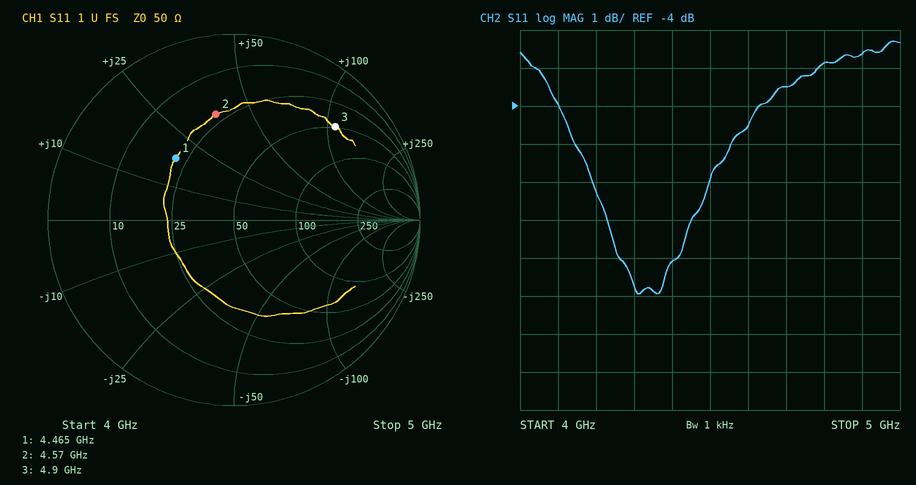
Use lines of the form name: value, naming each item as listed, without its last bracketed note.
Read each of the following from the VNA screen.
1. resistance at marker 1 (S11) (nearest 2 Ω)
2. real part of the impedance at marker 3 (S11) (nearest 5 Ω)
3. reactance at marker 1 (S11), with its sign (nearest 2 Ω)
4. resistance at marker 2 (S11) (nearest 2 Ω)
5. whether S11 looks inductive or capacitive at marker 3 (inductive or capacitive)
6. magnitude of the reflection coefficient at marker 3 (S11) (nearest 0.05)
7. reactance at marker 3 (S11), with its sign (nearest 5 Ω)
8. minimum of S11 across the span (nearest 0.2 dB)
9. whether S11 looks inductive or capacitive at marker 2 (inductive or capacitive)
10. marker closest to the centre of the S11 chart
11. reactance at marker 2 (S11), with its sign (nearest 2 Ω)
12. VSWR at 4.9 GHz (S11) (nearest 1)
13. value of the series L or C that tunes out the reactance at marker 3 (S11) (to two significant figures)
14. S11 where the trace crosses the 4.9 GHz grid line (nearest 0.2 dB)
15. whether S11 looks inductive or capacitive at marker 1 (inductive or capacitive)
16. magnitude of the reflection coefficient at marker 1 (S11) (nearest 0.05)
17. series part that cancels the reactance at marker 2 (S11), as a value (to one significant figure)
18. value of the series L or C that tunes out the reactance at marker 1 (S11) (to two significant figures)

resistance at marker 1 (S11): 22 Ω
real part of the impedance at marker 3 (S11): 50 Ω
reactance at marker 1 (S11), with its sign: +18 Ω
resistance at marker 2 (S11): 22 Ω
whether S11 looks inductive or capacitive at marker 3: inductive
magnitude of the reflection coefficient at marker 3 (S11): 0.75
reactance at marker 3 (S11), with its sign: +110 Ω
minimum of S11 across the span: -9.0 dB
whether S11 looks inductive or capacitive at marker 2: inductive
marker closest to the centre of the S11 chart: marker 1
reactance at marker 2 (S11), with its sign: +38 Ω
VSWR at 4.9 GHz (S11): 7
value of the series L or C that tunes out the reactance at marker 3 (S11): 300 fF
S11 where the trace crosses the 4.9 GHz grid line: -2.6 dB
whether S11 looks inductive or capacitive at marker 1: inductive
magnitude of the reflection coefficient at marker 1 (S11): 0.45
series part that cancels the reactance at marker 2 (S11), as a value: 900 fF
value of the series L or C that tunes out the reactance at marker 1 (S11): 2.0 pF
